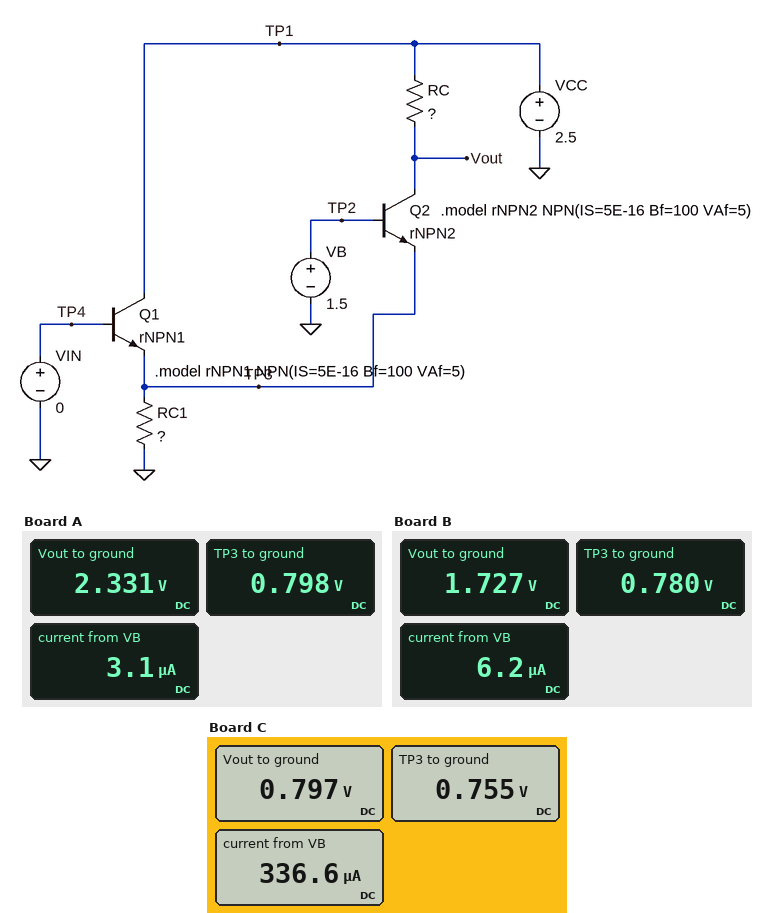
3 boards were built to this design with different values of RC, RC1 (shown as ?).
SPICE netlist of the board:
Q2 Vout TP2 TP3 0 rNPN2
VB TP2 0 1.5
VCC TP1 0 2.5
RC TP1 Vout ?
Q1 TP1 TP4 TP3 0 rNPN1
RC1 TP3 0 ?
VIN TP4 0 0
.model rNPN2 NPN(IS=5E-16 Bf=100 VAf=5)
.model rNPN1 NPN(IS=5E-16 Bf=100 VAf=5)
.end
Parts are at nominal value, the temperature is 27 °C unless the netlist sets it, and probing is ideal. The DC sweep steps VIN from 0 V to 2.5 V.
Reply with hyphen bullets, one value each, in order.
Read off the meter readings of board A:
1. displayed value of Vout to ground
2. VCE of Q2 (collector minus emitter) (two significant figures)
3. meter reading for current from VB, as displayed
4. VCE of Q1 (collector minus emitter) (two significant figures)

- 2.331 V
- 1.5 V
- 3.1 µA
- 1.7 V
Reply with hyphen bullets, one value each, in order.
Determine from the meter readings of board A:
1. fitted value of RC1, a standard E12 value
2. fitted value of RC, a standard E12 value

- 2.2 kΩ
- 470 Ω
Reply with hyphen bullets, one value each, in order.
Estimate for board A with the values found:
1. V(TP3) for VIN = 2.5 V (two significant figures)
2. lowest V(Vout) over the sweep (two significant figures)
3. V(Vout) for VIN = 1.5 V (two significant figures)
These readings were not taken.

- 1.8 V
- 2.3 V
- 2.4 V
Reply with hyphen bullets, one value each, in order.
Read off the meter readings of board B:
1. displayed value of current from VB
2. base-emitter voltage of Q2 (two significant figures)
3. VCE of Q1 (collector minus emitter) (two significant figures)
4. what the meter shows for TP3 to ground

- 6.2 µA
- 720 mV
- 1.7 V
- 0.780 V
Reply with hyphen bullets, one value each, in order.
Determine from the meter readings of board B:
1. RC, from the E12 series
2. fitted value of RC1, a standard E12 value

- 1.2 kΩ
- 1.2 kΩ
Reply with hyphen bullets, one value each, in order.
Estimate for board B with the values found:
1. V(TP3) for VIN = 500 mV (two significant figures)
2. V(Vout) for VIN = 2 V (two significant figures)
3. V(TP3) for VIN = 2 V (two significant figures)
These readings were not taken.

- 780 mV
- 2.5 V
- 1.3 V
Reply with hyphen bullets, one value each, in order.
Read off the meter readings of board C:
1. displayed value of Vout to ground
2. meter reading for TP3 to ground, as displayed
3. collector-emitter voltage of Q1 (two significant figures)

- 0.797 V
- 0.755 V
- 1.7 V
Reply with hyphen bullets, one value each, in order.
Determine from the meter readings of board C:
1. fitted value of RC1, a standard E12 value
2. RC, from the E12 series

- 680 Ω
- 2.2 kΩ
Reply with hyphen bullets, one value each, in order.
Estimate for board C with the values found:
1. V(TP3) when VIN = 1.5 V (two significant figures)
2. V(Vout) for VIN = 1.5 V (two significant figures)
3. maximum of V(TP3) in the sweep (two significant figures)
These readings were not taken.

- 780 mV
- 1.4 V
- 1.7 V
